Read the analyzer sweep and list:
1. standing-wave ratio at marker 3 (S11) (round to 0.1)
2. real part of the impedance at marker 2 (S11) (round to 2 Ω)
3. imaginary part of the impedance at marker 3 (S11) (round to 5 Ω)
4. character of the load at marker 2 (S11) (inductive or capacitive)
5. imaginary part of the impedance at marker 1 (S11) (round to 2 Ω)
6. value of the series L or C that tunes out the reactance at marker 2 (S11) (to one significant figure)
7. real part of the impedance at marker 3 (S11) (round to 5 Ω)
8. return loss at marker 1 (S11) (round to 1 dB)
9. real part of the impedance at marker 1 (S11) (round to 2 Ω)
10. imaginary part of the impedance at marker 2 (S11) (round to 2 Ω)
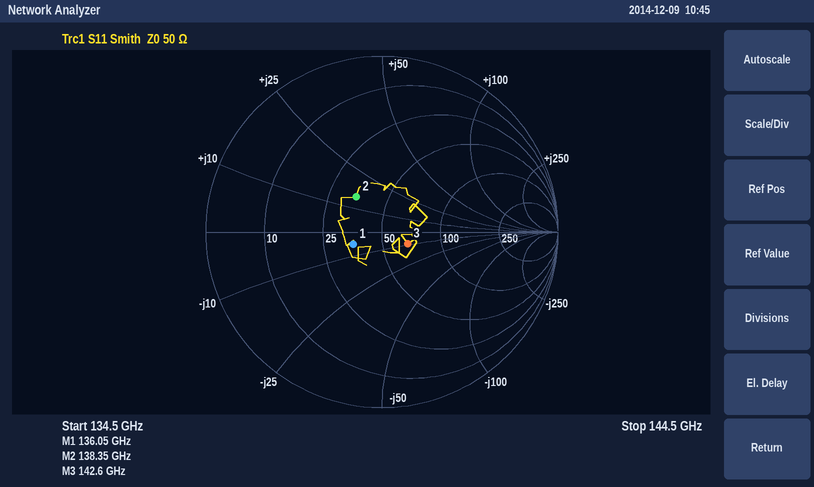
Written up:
1.4
34 Ω
-10 Ω
inductive
-6 Ω
80 fF
65 Ω
15 dB
36 Ω
+14 Ω
